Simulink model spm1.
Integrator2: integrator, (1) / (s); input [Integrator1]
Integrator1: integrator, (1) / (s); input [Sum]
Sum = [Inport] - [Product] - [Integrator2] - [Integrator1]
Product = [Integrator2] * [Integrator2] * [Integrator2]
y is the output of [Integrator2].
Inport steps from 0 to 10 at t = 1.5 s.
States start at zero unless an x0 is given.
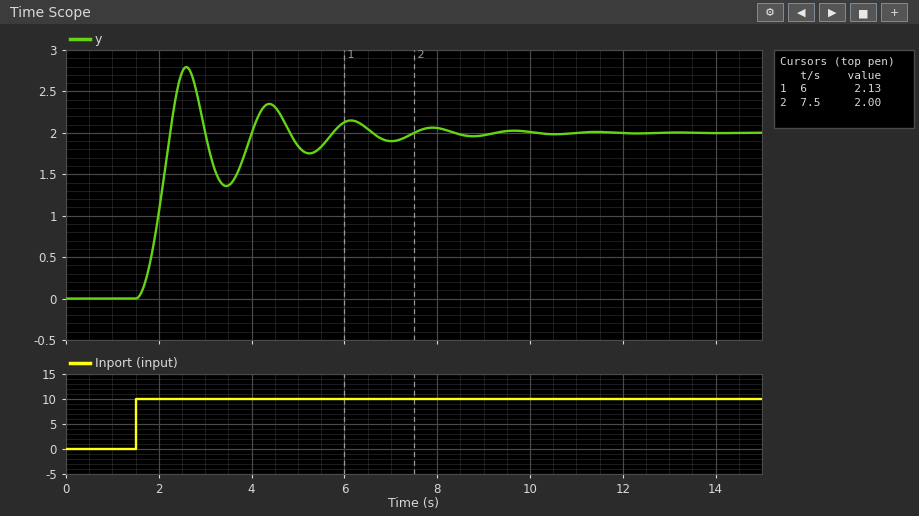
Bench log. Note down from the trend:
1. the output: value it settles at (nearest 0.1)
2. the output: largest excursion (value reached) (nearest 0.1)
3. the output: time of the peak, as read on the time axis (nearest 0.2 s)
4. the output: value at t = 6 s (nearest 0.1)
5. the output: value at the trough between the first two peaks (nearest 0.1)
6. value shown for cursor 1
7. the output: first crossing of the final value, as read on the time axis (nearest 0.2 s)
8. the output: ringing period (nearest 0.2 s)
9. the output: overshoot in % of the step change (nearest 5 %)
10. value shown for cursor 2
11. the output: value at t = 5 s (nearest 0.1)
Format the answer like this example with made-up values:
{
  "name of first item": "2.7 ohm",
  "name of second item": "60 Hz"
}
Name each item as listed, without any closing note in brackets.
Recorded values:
{
  "the output: value it settles at": "2.0",
  "the output: largest excursion (value reached)": "2.8",
  "the output: time of the peak, as read on the time axis": "2.6 s",
  "the output: value at t = 6 s": "2.1",
  "the output: value at the trough between the first two peaks": "1.4",
  "value shown for cursor 1": "2.13",
  "the output: first crossing of the final value, as read on the time axis": "2.2 s",
  "the output: ringing period": "1.8 s",
  "the output: overshoot in % of the step change": "40 %",
  "value shown for cursor 2": "2.00",
  "the output: value at t = 5 s": "1.8"
}
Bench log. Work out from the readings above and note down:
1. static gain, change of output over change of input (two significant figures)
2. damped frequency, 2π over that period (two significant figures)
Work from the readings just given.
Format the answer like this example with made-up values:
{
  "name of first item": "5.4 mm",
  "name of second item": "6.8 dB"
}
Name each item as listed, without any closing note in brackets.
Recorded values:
{
  "static gain, change of output over change of input": "0.20",
  "damped frequency, 2π over that period": "3.5 rad/s"
}
